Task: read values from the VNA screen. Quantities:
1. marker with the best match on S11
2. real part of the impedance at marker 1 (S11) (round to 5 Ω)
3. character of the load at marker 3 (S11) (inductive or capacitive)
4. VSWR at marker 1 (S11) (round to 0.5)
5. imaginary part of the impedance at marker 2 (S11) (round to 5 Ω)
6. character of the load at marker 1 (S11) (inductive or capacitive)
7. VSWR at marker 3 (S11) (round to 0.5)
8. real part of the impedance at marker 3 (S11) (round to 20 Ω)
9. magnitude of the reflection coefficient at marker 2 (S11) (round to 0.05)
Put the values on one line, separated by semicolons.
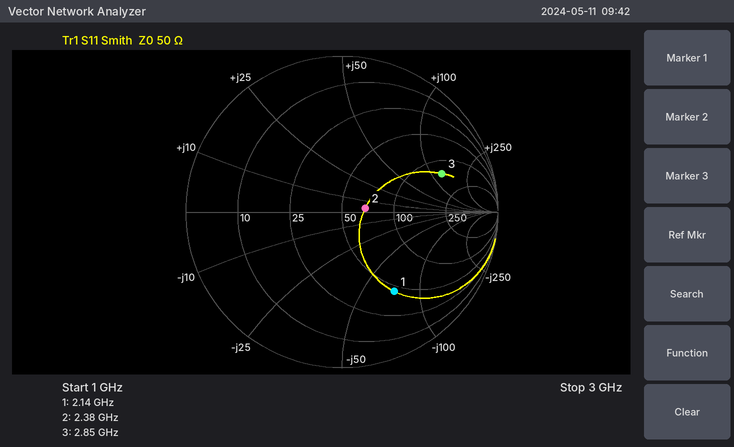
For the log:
marker 2; 45 Ω; inductive; 4.0; +5 Ω; capacitive; 5.5; 140 Ω; 0.15
